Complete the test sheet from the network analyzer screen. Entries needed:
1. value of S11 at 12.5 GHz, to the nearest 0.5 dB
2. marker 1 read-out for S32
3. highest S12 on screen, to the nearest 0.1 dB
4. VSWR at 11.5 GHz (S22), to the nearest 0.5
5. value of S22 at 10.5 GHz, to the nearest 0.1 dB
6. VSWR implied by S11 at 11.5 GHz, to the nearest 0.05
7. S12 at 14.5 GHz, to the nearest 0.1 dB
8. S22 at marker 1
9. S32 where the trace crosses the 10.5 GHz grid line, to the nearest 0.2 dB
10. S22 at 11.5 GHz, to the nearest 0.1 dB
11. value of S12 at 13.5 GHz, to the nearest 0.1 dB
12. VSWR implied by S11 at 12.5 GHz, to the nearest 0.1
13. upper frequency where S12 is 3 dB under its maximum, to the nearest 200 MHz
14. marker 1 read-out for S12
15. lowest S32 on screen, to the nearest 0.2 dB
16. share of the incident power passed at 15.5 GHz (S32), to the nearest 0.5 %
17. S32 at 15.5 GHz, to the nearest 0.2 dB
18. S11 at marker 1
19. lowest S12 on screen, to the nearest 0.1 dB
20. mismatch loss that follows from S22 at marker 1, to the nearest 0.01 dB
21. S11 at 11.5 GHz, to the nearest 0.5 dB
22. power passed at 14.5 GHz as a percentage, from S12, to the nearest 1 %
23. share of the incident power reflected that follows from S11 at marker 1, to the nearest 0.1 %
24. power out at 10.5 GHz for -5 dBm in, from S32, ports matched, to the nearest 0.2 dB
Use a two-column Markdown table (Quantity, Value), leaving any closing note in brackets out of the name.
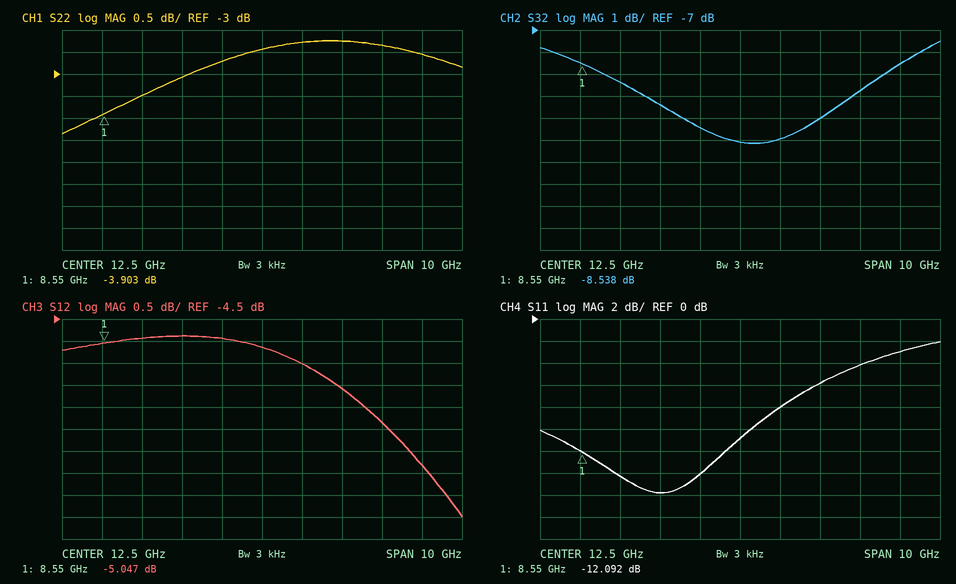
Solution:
| Quantity | Value |
|---|---|
| value of S11 at 12.5 GHz, to the nearest 0.5 dB | -11.0 dB |
| marker 1 read-out for S32 | -8.538 dB |
| highest S12 on screen, to the nearest 0.1 dB | -4.9 dB |
| VSWR at 11.5 GHz (S22), to the nearest 0.5 | 6.5 |
| value of S22 at 10.5 GHz, to the nearest 0.1 dB | -3.1 dB |
| VSWR implied by S11 at 11.5 GHz, to the nearest 0.05 | 1.50 |
| S12 at 14.5 GHz, to the nearest 0.1 dB | -6.1 dB |
| S22 at marker 1 | -3.903 dB |
| S32 where the trace crosses the 10.5 GHz grid line, to the nearest 0.2 dB | -10.4 dB |
| S22 at 11.5 GHz, to the nearest 0.1 dB | -2.7 dB |
| value of S12 at 13.5 GHz, to the nearest 0.1 dB | -5.5 dB |
| VSWR implied by S11 at 12.5 GHz, to the nearest 0.1 | 1.8 |
| upper frequency where S12 is 3 dB under its maximum, to the nearest 200 MHz | 16.6 GHz |
| marker 1 read-out for S12 | -5.047 dB |
| lowest S32 on screen, to the nearest 0.2 dB | -12.2 dB |
| share of the incident power passed at 15.5 GHz (S32), to the nearest 0.5 % | 10.5 % |
| S32 at 15.5 GHz, to the nearest 0.2 dB | -9.8 dB |
| S11 at marker 1 | -12.092 dB |
| lowest S12 on screen, to the nearest 0.1 dB | -9.0 dB |
| mismatch loss that follows from S22 at marker 1, to the nearest 0.01 dB | 2.27 dB |
| S11 at 11.5 GHz, to the nearest 0.5 dB | -14.0 dB |
| power passed at 14.5 GHz as a percentage, from S12, to the nearest 1 % | 25 % |
| share of the incident power reflected that follows from S11 at marker 1, to the nearest 0.1 % | 6.2 % |
| power out at 10.5 GHz for -5 dBm in, from S32, ports matched, to the nearest 0.2 dB | -15.4 dBm |
